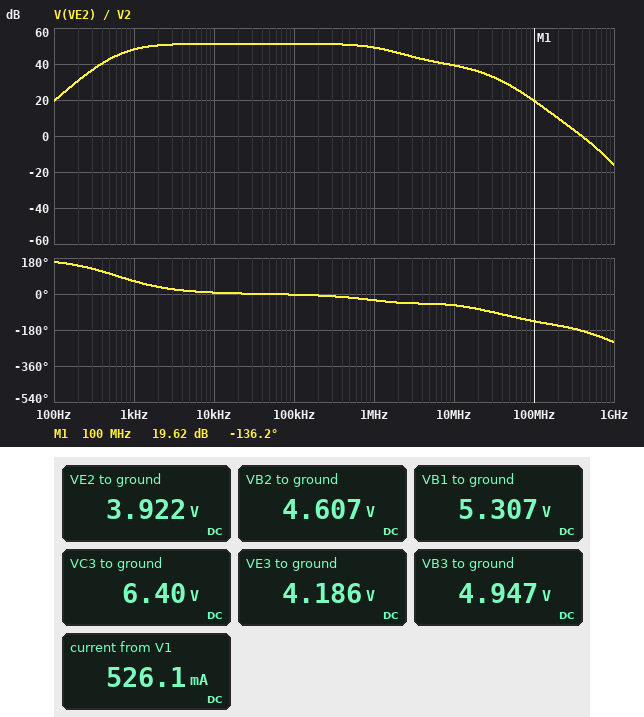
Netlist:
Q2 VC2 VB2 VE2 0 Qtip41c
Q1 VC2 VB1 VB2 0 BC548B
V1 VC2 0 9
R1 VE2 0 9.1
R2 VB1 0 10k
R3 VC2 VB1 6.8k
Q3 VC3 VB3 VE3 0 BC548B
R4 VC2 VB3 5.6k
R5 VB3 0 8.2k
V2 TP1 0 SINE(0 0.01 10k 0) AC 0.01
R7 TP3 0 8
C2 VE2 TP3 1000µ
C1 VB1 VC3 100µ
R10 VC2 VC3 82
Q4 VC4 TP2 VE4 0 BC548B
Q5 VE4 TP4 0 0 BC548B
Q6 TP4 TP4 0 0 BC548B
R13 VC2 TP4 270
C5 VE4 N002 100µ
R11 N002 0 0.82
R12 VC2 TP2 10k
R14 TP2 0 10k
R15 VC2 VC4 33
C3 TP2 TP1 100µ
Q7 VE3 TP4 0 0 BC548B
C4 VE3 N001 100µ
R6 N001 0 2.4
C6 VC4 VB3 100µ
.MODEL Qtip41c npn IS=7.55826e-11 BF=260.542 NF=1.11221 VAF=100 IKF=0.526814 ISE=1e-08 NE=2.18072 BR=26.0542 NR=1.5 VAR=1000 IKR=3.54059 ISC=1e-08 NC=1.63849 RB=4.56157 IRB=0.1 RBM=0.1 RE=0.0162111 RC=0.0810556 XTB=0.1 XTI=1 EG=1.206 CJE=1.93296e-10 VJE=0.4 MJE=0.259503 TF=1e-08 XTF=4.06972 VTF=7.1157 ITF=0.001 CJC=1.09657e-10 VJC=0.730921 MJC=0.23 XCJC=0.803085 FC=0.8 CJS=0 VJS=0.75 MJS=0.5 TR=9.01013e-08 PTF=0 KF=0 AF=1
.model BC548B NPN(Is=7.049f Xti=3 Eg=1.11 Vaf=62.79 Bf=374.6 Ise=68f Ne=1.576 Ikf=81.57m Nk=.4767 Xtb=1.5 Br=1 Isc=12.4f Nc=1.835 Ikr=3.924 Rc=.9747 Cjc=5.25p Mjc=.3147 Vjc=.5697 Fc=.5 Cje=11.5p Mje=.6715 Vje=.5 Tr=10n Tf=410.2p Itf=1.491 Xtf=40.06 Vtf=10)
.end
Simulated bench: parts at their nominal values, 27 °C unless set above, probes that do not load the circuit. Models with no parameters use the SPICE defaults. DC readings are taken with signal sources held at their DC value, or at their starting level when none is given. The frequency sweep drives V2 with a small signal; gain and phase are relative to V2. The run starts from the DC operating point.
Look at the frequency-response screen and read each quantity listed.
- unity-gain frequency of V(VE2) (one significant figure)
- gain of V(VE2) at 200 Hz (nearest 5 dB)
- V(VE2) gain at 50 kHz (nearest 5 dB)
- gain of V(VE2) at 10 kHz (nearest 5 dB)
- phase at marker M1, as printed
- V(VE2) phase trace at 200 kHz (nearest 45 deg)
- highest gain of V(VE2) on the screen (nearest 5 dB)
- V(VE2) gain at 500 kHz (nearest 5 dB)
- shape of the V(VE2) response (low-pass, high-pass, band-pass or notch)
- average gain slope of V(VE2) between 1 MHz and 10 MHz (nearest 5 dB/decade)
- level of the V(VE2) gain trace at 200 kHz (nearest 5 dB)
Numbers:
400 MHz
30 dB
50 dB
50 dB
-136.2 deg
0 deg
50 dB
50 dB
band-pass
-10 dB/decade
50 dB
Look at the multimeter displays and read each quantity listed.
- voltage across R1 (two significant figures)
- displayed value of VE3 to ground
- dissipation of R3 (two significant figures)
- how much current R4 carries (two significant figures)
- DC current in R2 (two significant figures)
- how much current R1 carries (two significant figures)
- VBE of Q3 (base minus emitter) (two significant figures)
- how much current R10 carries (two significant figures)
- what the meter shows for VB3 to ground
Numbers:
3.9 V
4.186 V
2.0 mW
720 µA
530 µA
430 mA
760 mV
32 mA
4.947 V
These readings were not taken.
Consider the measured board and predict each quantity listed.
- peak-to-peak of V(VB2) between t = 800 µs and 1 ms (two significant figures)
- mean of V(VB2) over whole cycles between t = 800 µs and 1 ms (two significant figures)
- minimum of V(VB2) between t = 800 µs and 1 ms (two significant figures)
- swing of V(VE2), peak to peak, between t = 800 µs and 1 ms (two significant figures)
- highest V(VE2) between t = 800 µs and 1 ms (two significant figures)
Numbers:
4.4 V
4.7 V
2.7 V
4.1 V
6.3 V
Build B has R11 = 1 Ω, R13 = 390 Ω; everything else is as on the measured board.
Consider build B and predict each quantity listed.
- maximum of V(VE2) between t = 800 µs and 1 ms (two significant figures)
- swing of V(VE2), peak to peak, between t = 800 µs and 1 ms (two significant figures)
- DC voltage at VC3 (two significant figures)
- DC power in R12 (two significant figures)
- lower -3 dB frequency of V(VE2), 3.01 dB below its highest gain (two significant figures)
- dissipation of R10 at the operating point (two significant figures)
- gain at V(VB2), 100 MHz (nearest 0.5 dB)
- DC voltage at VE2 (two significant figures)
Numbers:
5.6 V
3.5 V
7.2 V
2.4 mW
840 Hz
40 mW
24.0 dB
3.9 V
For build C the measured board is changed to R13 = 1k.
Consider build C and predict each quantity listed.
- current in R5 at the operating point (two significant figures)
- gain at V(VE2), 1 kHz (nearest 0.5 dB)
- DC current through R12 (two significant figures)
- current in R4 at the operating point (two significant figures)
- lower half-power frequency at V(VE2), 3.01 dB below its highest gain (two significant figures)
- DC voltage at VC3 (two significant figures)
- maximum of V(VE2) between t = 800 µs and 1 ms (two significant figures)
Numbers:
640 µA
39.5 dB
460 µA
670 µA
520 Hz
8.3 V
4.5 V
